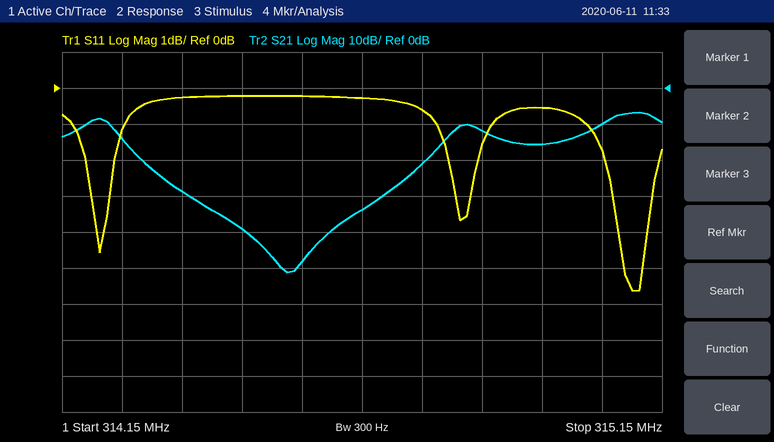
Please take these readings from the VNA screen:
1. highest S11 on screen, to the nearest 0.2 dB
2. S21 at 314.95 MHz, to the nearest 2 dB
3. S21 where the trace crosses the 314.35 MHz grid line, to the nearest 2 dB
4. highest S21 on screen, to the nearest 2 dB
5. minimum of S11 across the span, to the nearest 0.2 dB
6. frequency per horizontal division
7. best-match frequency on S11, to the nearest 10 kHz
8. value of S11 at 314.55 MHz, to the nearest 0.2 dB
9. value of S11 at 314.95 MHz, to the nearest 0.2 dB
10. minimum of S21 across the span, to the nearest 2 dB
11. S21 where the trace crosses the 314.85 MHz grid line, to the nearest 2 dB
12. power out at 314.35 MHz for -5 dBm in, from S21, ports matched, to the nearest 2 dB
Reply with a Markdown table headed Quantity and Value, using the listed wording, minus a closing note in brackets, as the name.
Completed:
| Quantity | Value |
|---|---|
| highest S11 on screen, to the nearest 0.2 dB | -0.2 dB |
| S21 at 314.95 MHz, to the nearest 2 dB | -16 dB |
| S21 where the trace crosses the 314.35 MHz grid line, to the nearest 2 dB | -28 dB |
| highest S21 on screen, to the nearest 2 dB | -6 dB |
| minimum of S11 across the span, to the nearest 0.2 dB | -5.6 dB |
| frequency per horizontal division | 100 kHz |
| best-match frequency on S11, to the nearest 10 kHz | 315.10 MHz |
| value of S11 at 314.55 MHz, to the nearest 0.2 dB | -0.2 dB |
| value of S11 at 314.95 MHz, to the nearest 0.2 dB | -0.6 dB |
| minimum of S21 across the span, to the nearest 2 dB | -52 dB |
| S21 where the trace crosses the 314.85 MHz grid line, to the nearest 2 dB | -12 dB |
| power out at 314.35 MHz for -5 dBm in, from S21, ports matched, to the nearest 2 dB | -34 dBm |
